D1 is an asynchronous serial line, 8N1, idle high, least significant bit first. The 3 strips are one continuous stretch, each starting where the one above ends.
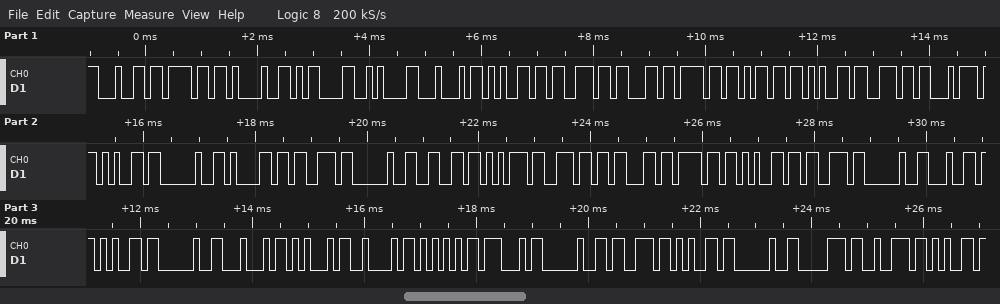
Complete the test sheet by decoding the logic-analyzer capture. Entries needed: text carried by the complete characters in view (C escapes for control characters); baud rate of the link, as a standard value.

"do!\r\nDescomente as funcoes de DEBUG se pre"
9600 baud
